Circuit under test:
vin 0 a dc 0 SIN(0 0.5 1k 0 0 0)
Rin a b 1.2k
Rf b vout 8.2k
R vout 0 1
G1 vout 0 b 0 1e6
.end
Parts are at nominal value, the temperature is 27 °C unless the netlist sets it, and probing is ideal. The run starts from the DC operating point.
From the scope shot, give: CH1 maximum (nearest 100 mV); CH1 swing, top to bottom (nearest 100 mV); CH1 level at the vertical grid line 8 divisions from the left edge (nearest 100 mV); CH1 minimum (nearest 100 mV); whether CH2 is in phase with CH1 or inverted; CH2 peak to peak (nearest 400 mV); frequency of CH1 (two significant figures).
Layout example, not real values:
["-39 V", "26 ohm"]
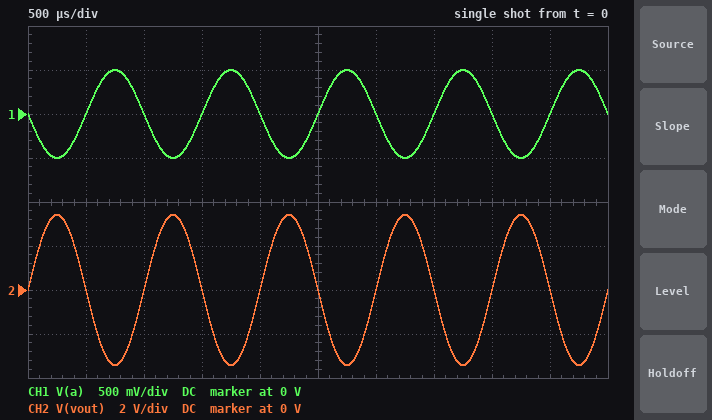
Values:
["500 mV", "1.0 V", "0 V", "-500 mV", "inverted", "6.8 V", "1.0 kHz"]
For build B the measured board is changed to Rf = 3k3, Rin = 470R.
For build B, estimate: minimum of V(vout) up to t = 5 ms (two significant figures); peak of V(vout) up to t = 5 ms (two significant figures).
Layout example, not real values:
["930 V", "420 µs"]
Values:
["-3.5 V", "3.5 V"]
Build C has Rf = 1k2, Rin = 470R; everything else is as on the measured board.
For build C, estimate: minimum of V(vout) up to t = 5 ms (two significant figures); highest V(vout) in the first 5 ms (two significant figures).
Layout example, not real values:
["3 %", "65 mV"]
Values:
["-1.3 V", "1.3 V"]
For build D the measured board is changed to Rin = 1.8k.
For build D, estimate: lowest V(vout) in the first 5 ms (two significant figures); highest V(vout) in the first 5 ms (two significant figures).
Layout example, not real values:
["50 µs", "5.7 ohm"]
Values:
["-2.3 V", "2.3 V"]
